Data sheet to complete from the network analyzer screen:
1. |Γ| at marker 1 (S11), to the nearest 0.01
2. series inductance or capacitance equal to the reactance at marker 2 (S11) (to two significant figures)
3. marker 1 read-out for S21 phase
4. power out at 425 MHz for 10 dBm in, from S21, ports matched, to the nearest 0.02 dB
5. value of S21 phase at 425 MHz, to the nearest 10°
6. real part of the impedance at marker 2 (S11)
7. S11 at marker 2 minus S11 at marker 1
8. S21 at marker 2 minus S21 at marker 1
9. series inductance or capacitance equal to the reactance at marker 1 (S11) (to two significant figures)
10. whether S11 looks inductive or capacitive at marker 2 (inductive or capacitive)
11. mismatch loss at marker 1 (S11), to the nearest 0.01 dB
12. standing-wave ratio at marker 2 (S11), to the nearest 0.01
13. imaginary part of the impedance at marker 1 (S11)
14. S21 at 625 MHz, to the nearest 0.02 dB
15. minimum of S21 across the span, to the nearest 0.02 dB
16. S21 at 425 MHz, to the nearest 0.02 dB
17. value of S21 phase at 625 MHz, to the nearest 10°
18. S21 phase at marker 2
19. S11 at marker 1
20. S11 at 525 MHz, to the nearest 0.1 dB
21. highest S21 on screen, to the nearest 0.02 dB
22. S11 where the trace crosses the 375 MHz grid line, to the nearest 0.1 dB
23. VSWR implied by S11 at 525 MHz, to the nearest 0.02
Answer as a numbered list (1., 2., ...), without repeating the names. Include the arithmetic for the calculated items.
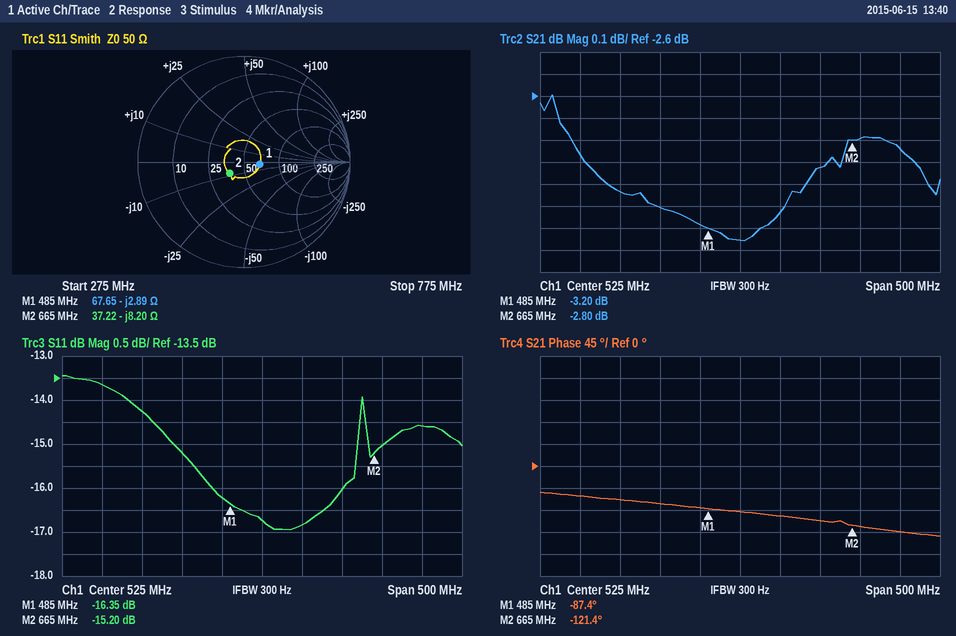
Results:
1. 0.15
2. C = 1/(2π × 665 MHz × 8.2 Ω) ≈ 29 pF
3. -87.4°
4. 10 dBm + (-3.10 dB) = 6.90 dBm
5. -80°
6. 37.22 Ω
7. -15.2 − (-16.35) = 1.15 dB
8. -2.8 − (-3.2) = 0.40 dB
9. C = 1/(2π × 485 MHz × 2.89 Ω) ≈ 114 pF, so 110 pF to two significant figures
10. capacitive
11. −10 log10(1 − 10^(-16.35/10)) ≈ 0.10 dB
12. 1.42
13. -2.89 Ω
14. -2.92 dB
15. -3.26 dB
16. -3.10 dB
17. -110°
18. -121.4°
19. -16.35 dB
20. -16.7 dB
21. -2.60 dB
22. -14.3 dB
23. |Γ| = 10^(-16.7/20) = 0.1462; VSWR = (1 + 0.1462)/(1 − 0.1462) ≈ 1.34
